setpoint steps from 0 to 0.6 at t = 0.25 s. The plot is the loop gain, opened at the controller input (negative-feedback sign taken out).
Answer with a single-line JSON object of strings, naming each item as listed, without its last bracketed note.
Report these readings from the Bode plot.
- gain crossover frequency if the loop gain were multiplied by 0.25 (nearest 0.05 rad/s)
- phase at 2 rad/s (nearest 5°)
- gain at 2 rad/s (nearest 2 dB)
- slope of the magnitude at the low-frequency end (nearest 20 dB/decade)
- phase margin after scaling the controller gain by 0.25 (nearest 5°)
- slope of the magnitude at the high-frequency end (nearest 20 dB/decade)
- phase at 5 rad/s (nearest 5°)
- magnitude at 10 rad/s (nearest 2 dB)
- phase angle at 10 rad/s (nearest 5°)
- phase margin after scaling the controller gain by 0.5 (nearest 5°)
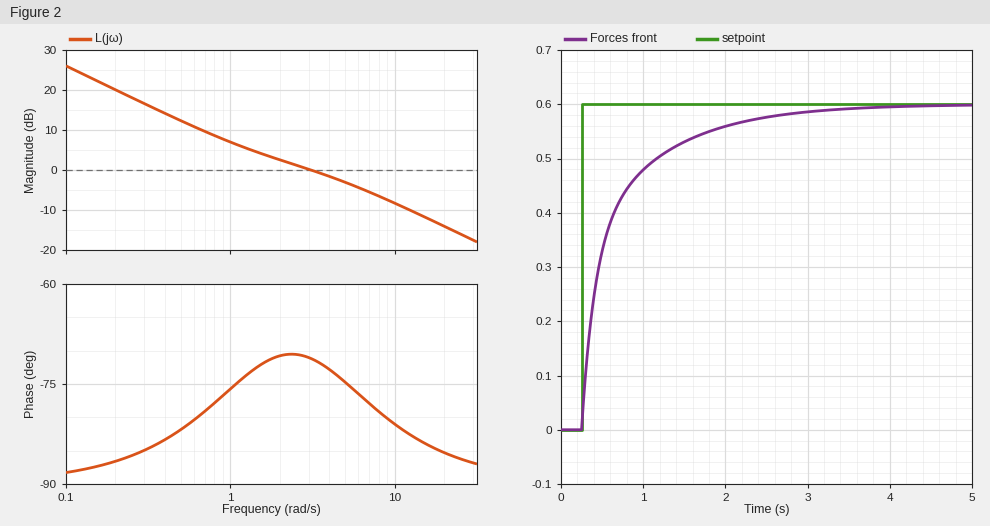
{"gain crossover frequency if the loop gain were multiplied by 0.25": "0.50 rad/s", "phase at 2 rad/s": "-70°", "gain at 2 rad/s": "2 dB", "slope of the magnitude at the low-frequency end": "-20 dB/decade", "phase margin after scaling the controller gain by 0.25": "100°", "slope of the magnitude at the high-frequency end": "-20 dB/decade", "phase at 5 rad/s": "-75°", "magnitude at 10 rad/s": "-8 dB", "phase angle at 10 rad/s": "-80°", "phase margin after scaling the controller gain by 0.5": "105°"}
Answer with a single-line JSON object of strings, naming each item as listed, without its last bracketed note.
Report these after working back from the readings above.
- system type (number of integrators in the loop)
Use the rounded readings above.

{"system type": "1"}
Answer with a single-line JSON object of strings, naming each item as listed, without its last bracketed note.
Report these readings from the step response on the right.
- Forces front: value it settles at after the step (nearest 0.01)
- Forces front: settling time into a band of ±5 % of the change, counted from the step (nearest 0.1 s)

{"Forces front: value it settles at after the step": "0.60", "Forces front: settling time into a band of ±5 % of the change, counted from the step": "2.0 s"}
